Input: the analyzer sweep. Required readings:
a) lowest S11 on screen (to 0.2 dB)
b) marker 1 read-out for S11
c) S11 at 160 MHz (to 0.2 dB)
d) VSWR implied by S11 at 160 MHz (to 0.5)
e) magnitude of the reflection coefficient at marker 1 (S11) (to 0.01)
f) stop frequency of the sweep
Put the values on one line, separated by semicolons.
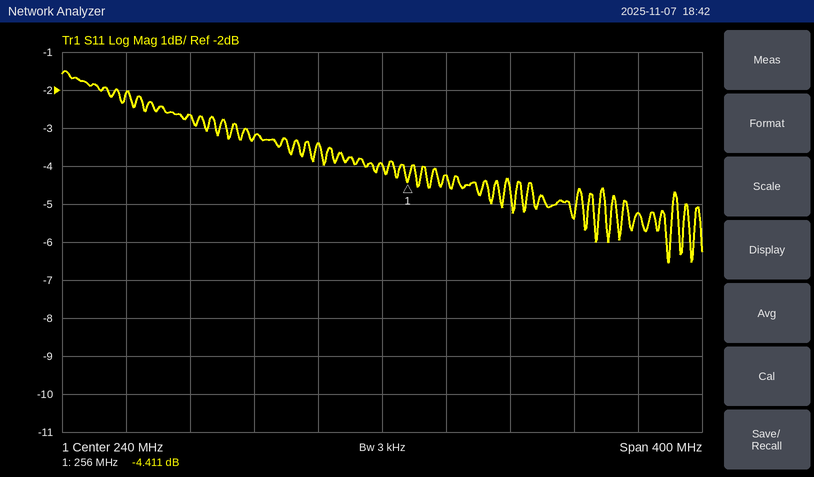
-6.6 dB; -4.411 dB; -3.2 dB; 5.5; 0.60; 440 MHz
